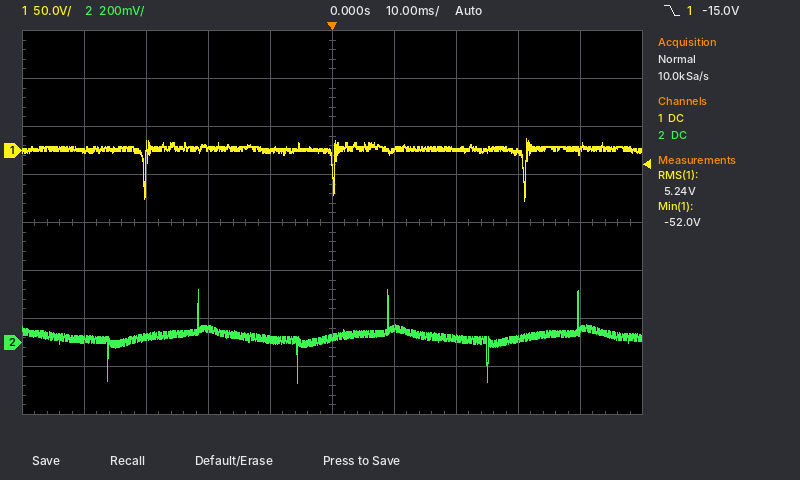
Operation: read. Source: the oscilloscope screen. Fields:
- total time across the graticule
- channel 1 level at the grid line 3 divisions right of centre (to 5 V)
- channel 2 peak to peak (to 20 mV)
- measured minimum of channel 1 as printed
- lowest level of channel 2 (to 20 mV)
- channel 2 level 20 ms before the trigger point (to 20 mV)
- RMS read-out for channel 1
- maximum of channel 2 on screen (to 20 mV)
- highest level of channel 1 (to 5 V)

100 ms
0 V
380 mV
-52.0 V
-160 mV
60 mV
5.24 V
220 mV
10 V
